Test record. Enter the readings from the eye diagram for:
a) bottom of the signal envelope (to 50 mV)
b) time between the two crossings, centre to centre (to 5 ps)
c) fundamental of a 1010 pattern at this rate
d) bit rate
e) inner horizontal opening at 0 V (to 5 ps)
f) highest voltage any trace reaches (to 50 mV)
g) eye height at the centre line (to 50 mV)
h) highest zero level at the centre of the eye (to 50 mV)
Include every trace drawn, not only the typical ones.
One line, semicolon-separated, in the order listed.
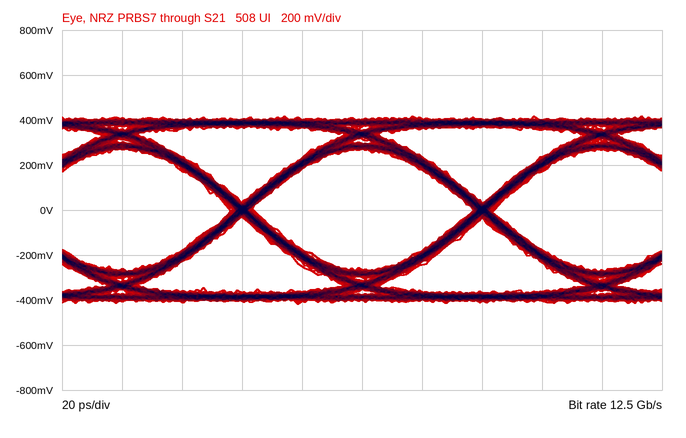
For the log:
-400 mV; 80 ps; 6.25 GHz; 12.5 Gb/s; 75 ps; 400 mV; 550 mV; -250 mV
